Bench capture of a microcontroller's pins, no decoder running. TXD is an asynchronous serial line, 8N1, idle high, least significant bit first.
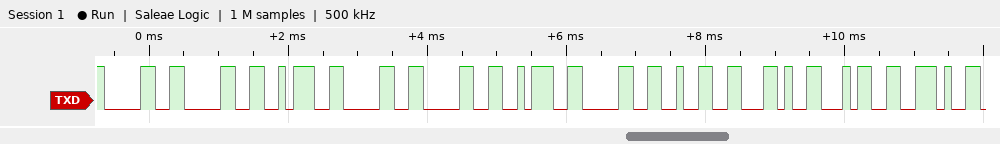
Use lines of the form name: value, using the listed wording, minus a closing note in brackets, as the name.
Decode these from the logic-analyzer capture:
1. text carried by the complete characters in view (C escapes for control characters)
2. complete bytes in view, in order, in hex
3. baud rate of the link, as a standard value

text carried by the complete characters in view: "00:00:02,4."
complete bytes in view, in order, in hex: 30 30 3A 30 30 3A 30 32 2C 34 2E
baud rate of the link, as a standard value: 9600 baud
